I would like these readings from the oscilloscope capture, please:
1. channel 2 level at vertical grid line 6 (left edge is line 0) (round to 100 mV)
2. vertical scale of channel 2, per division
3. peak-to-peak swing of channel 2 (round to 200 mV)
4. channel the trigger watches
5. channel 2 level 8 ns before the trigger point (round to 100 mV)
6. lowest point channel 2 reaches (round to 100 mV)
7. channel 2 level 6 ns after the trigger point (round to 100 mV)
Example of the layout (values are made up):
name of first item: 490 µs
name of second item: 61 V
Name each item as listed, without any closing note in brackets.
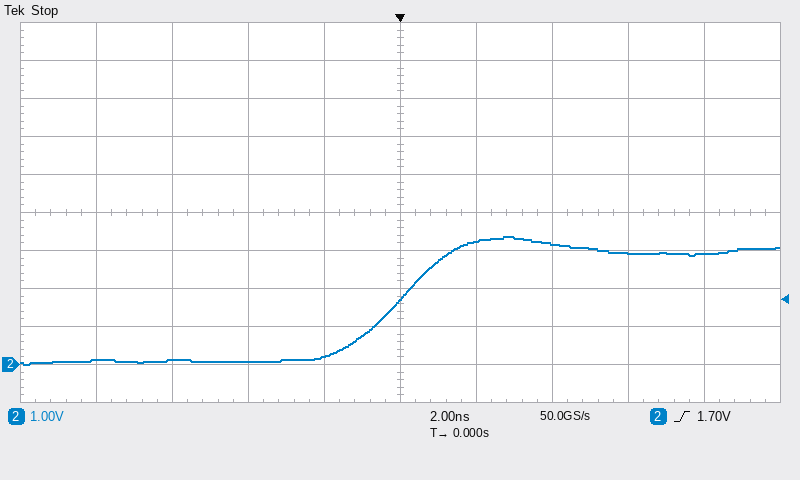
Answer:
channel 2 level at vertical grid line 6 (left edge is line 0): 3.2 V
vertical scale of channel 2, per division: 1 V
peak-to-peak swing of channel 2: 3.4 V
channel the trigger watches: channel 2
channel 2 level 8 ns before the trigger point: 100 mV
lowest point channel 2 reaches: 0.0 V
channel 2 level 6 ns after the trigger point: 2.9 V
